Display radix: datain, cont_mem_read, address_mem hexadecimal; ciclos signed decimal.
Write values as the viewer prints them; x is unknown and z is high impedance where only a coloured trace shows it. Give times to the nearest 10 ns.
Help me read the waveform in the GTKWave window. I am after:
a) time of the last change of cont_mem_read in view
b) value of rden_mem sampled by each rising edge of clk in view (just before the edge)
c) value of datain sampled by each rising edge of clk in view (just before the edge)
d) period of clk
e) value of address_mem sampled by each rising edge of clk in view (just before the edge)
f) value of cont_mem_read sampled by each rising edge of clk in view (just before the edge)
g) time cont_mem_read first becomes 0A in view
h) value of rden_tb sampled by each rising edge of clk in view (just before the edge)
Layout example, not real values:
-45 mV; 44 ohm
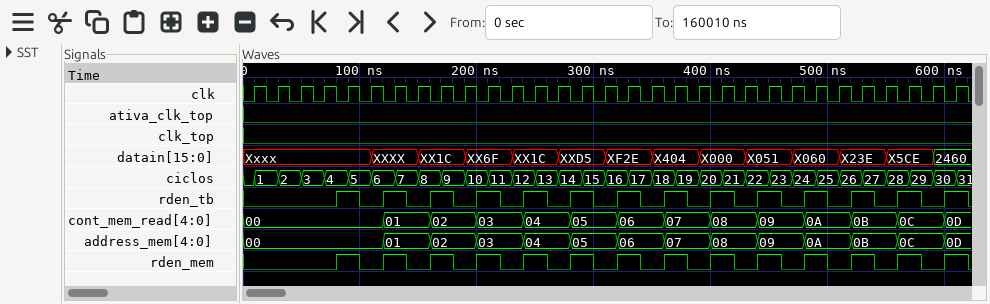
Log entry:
600 ns; 0 0 0 0 1 0 1 0 1 0 1 0 1 0 1 0 1 0 1 0 1 0 1 0 1 0 1 0 1 0 1; Xxxx, Xxxx, Xxxx, Xxxx, Xxxx, Xxxx, XXXX, XXXX, XX1C, XX1C, XX6F, XX6F, XX1C, XX1C, XXD5, XXD5, XF2E, XF2E, X404, X404, X000, X000, X051, X051, X060, X060, X23E, X23E, X5CE, X5CE, 2460; 20 ns; 00, 00, 00, 00, 00, 00, 01, 01, 02, 02, 03, 03, 04, 04, 05, 05, 06, 06, 07, 07, 08, 08, 09, 09, 0A, 0A, 0B, 0B, 0C, 0C, 0D; 00, 00, 00, 00, 00, 00, 01, 01, 02, 02, 03, 03, 04, 04, 05, 05, 06, 06, 07, 07, 08, 08, 09, 09, 0A, 0A, 0B, 0B, 0C, 0C, 0D; 480 ns; 0 0 0 0 1 0 1 0 1 0 1 0 1 0 1 0 1 0 1 0 1 0 1 0 1 0 1 0 1 0 1
